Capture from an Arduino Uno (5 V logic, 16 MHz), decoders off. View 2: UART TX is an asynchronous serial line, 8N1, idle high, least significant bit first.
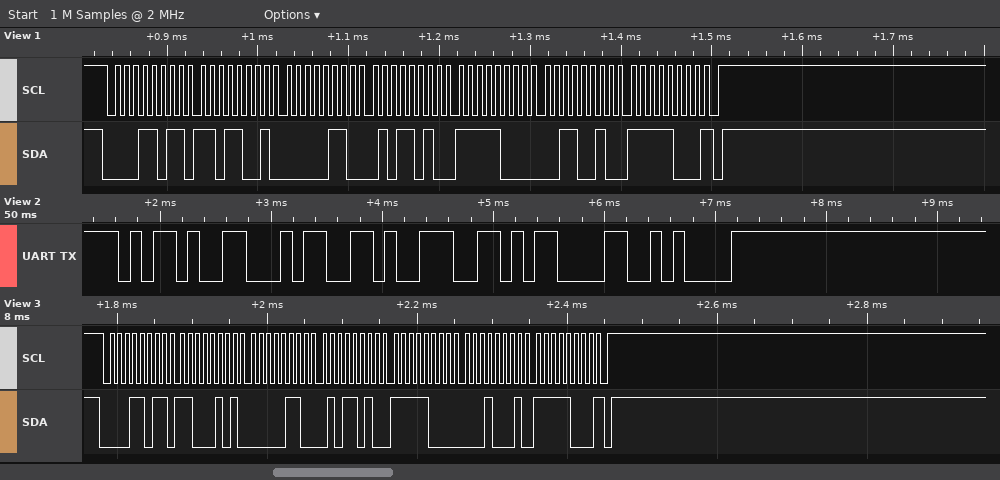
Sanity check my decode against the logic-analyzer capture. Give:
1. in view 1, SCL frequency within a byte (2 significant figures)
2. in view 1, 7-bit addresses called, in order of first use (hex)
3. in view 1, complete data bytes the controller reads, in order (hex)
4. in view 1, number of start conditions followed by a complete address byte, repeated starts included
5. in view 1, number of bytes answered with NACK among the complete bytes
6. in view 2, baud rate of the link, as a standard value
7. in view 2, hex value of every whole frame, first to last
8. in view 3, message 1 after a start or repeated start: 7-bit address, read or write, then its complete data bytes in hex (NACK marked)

100 kHz
0x0D
D9 06 5A F8 32 F8
1
1
9600 baud
0x2D 0x34 0x39 0x0D 0x0A
0x0D read: C5 06 5A F8 11 F8 NACK
